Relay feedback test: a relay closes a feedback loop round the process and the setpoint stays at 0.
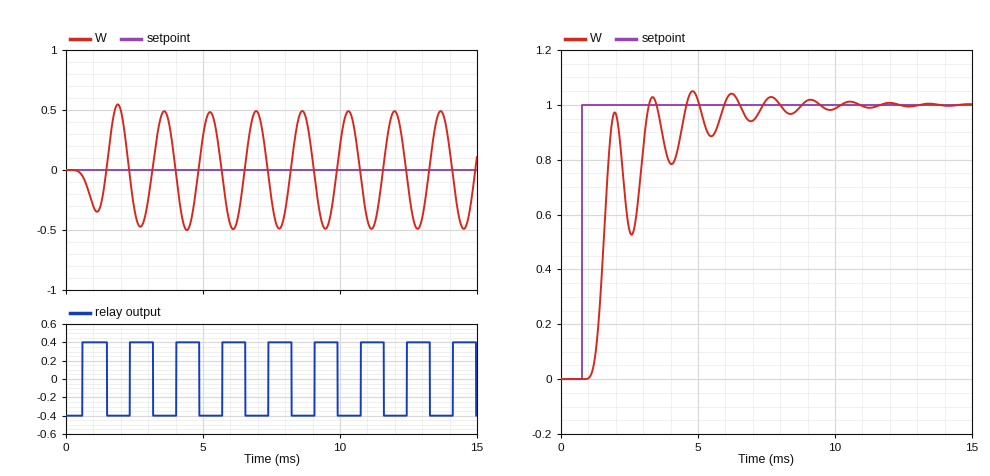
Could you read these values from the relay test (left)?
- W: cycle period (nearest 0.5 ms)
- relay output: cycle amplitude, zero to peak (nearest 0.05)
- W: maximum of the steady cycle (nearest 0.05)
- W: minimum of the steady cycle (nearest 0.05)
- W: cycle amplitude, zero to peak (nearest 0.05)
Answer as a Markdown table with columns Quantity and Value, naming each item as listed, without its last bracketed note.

| Quantity | Value |
|---|---|
| W: cycle period | 1.5 ms |
| relay output: cycle amplitude, zero to peak | 0.40 |
| W: maximum of the steady cycle | 0.50 |
| W: minimum of the steady cycle | -0.50 |
| W: cycle amplitude, zero to peak | 0.50 |
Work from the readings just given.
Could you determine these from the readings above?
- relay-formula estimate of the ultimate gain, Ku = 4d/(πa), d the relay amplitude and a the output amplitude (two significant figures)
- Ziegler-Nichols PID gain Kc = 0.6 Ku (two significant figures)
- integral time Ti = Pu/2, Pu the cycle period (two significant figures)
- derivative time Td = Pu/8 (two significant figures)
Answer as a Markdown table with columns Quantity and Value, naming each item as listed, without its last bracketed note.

| Quantity | Value |
|---|---|
| relay-formula estimate of the ultimate gain, Ku = 4d/(πa), d the relay amplitude and a the output amplitude | 1.0 |
| Ziegler-Nichols PID gain Kc = 0.6 Ku | 0.60 |
| integral time Ti = Pu/2, Pu the cycle period | 0.75 ms |
| derivative time Td = Pu/8 | 0.19 ms |
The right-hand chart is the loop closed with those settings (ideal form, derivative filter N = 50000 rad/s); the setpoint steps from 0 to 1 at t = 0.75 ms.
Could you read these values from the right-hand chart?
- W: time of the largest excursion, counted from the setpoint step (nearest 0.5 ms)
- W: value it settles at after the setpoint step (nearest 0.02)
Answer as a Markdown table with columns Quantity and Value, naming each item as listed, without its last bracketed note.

| Quantity | Value |
|---|---|
| W: time of the largest excursion, counted from the setpoint step | 4.0 ms |
| W: value it settles at after the setpoint step | 1.00 |
